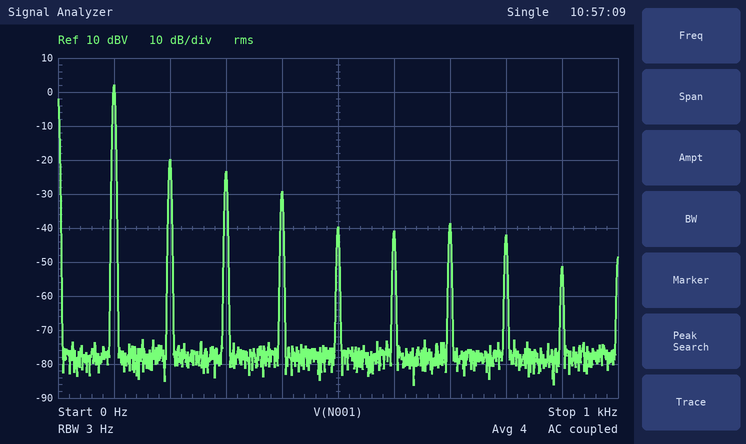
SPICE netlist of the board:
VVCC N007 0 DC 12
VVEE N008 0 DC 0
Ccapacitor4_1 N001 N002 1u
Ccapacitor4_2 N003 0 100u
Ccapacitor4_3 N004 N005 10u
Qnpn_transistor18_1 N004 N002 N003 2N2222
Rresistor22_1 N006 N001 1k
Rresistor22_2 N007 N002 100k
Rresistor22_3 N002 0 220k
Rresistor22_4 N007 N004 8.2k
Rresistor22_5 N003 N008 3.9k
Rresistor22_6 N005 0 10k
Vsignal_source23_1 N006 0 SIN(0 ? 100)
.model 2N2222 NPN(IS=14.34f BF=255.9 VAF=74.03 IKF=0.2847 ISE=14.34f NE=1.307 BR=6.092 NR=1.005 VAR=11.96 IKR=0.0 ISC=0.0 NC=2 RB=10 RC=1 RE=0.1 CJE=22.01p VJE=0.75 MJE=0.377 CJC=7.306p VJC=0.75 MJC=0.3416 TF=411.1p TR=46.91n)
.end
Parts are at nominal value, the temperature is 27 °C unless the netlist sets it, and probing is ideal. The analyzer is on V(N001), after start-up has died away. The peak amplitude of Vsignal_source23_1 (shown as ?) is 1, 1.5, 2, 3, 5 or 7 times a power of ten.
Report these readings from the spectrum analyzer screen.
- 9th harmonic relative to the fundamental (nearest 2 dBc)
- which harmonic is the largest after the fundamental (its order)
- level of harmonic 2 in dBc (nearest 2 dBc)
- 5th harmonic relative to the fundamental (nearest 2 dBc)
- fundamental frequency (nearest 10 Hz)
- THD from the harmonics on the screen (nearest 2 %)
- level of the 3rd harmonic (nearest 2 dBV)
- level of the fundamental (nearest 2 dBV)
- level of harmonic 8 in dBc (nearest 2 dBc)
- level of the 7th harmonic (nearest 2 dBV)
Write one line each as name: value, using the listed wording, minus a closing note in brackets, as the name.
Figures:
9th harmonic relative to the fundamental: -54 dBc
which harmonic is the largest after the fundamental: 2
level of harmonic 2 in dBc: -22 dBc
5th harmonic relative to the fundamental: -42 dBc
fundamental frequency: 100 Hz
THD from the harmonics on the screen: 10 %
level of the 3rd harmonic: -24 dBV
level of the fundamental: 2 dBV
level of harmonic 8 in dBc: -44 dBc
level of the 7th harmonic: -38 dBV
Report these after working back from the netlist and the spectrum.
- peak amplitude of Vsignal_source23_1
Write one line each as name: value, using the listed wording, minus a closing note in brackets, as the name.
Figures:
peak amplitude of Vsignal_source23_1: 2 V
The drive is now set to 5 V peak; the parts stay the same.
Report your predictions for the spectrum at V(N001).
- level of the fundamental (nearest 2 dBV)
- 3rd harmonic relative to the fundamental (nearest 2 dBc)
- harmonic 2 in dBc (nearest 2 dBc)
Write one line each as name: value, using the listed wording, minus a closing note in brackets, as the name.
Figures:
level of the fundamental: 10 dBV
3rd harmonic relative to the fundamental: -28 dBc
harmonic 2 in dBc: -26 dBc
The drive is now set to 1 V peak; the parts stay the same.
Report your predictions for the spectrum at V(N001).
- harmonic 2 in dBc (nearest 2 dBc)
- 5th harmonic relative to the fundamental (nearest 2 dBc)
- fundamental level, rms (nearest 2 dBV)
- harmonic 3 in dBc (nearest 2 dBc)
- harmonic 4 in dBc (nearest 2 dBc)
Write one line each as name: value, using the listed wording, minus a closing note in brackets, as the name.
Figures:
harmonic 2 in dBc: -18 dBc
5th harmonic relative to the fundamental: -38 dBc
fundamental level, rms: -4 dBV
harmonic 3 in dBc: -24 dBc
harmonic 4 in dBc: -36 dBc
